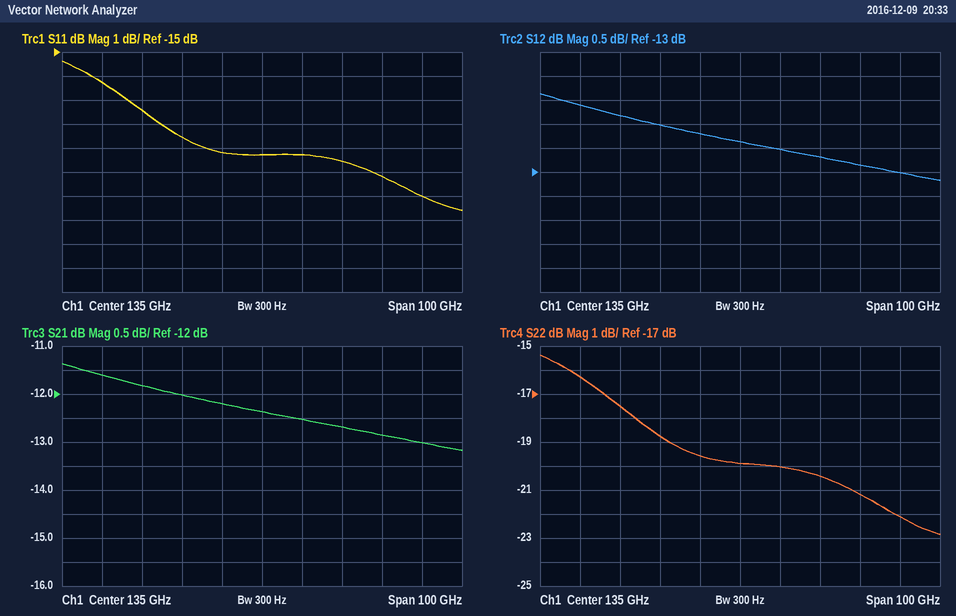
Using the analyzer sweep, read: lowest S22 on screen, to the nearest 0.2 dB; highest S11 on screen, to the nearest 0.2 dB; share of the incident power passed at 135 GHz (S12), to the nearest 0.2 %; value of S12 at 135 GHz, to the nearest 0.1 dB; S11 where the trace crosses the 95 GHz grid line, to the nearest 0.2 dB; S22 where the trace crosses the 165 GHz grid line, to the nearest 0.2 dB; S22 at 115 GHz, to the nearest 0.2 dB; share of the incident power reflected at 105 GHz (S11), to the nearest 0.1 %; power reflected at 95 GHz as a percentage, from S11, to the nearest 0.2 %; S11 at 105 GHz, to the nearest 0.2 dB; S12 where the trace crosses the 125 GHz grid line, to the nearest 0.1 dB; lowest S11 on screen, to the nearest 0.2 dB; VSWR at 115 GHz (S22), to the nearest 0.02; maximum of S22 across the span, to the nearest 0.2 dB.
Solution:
-22.8 dB
-15.4 dB
5.8 %
-12.4 dB
-16.2 dB
-21.2 dB
-18.8 dB
1.8 %
2.4 %
-17.4 dB
-12.2 dB
-21.6 dB
1.26
-15.4 dB
